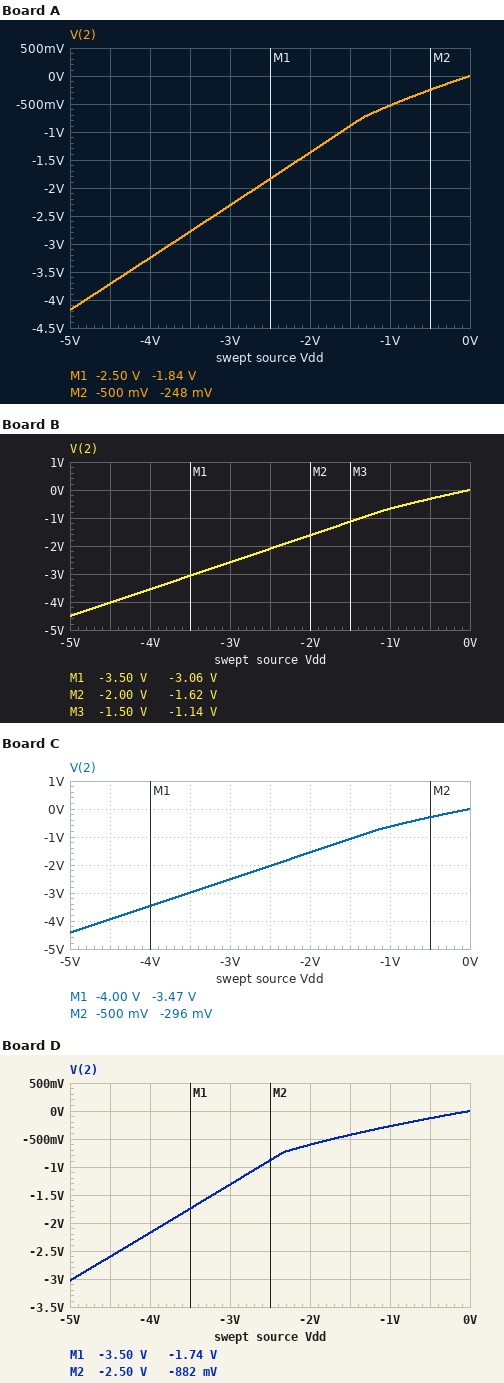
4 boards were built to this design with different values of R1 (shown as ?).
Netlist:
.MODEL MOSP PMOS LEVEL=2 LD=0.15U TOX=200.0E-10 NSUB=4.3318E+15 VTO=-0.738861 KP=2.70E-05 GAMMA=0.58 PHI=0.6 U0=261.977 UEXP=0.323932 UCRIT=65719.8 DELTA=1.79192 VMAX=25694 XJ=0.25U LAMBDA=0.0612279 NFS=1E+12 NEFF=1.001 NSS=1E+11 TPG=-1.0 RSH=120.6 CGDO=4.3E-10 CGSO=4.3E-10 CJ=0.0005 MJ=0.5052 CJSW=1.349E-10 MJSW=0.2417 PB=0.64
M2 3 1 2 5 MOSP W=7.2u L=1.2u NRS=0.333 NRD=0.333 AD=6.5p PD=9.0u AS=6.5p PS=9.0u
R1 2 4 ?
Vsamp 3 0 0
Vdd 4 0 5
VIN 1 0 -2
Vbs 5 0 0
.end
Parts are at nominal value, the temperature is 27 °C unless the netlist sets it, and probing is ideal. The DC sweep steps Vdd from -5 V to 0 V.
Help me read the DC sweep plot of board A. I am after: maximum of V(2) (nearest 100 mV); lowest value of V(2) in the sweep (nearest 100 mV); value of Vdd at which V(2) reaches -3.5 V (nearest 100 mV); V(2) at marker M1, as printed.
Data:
0 V
-4.2 V
-4.3 V
-1.84 V
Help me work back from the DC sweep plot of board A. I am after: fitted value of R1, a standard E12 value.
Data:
5.6 kΩ
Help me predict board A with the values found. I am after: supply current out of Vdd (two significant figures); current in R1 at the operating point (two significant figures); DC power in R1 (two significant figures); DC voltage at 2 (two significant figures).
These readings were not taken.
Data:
770 µA
770 µA
3.3 mW
670 mV
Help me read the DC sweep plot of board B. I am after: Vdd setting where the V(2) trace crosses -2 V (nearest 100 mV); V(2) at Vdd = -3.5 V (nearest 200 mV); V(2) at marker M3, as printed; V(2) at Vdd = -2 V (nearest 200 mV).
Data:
-2.4 V
-3.0 V
-1.14 V
-1.6 V
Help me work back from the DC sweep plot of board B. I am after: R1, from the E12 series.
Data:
3.3 kΩ
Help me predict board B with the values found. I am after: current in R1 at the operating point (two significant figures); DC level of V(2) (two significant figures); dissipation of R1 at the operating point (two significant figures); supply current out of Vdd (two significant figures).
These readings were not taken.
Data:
1.3 mA
710 mV
5.6 mW
1.3 mA
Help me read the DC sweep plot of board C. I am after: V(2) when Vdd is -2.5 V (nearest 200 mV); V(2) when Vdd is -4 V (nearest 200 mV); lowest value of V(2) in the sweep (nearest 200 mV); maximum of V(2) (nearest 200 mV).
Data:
-2.0 V
-3.4 V
-4.4 V
0 V
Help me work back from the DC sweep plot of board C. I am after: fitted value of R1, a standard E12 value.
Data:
3.9 kΩ
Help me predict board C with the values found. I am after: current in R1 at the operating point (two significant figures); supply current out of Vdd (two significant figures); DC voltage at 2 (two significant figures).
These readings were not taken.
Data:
1.1 mA
1.1 mA
700 mV
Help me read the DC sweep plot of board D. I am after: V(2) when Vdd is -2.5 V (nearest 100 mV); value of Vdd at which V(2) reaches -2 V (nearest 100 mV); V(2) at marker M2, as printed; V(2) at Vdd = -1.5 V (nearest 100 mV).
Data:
-900 mV
-3.8 V
-882 mV
-400 mV
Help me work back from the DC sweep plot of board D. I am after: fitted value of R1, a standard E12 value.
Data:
15 kΩ
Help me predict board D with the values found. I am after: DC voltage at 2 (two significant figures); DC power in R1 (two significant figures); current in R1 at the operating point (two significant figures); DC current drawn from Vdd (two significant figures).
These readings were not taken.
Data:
620 mV
1.3 mW
290 µA
290 µA
